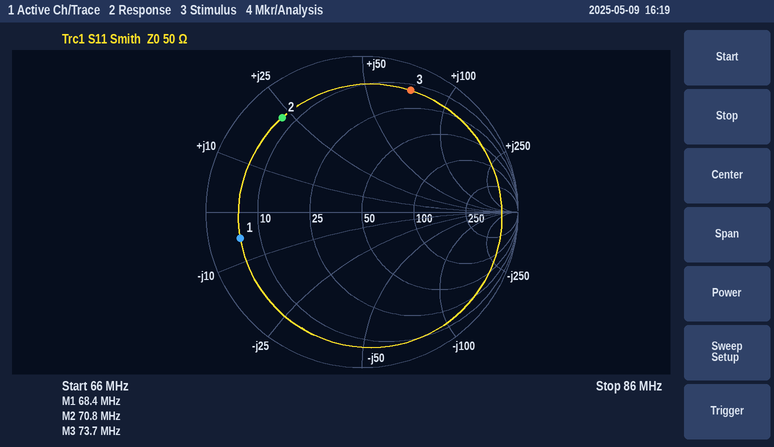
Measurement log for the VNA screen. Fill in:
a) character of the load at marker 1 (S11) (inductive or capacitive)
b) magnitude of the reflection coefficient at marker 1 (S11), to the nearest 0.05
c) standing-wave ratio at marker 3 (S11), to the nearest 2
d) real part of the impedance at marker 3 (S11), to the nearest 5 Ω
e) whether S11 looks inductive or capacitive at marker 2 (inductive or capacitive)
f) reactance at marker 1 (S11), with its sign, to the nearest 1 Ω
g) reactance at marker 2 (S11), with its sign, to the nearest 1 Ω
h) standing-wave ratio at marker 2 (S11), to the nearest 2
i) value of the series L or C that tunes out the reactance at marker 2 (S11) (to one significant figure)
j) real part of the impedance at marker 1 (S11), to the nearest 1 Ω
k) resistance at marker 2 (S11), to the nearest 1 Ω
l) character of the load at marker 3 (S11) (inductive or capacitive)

capacitive
0.80
12
15 Ω
inductive
-5 Ω
+23 Ω
8
100 pF
6 Ω
7 Ω
inductive
